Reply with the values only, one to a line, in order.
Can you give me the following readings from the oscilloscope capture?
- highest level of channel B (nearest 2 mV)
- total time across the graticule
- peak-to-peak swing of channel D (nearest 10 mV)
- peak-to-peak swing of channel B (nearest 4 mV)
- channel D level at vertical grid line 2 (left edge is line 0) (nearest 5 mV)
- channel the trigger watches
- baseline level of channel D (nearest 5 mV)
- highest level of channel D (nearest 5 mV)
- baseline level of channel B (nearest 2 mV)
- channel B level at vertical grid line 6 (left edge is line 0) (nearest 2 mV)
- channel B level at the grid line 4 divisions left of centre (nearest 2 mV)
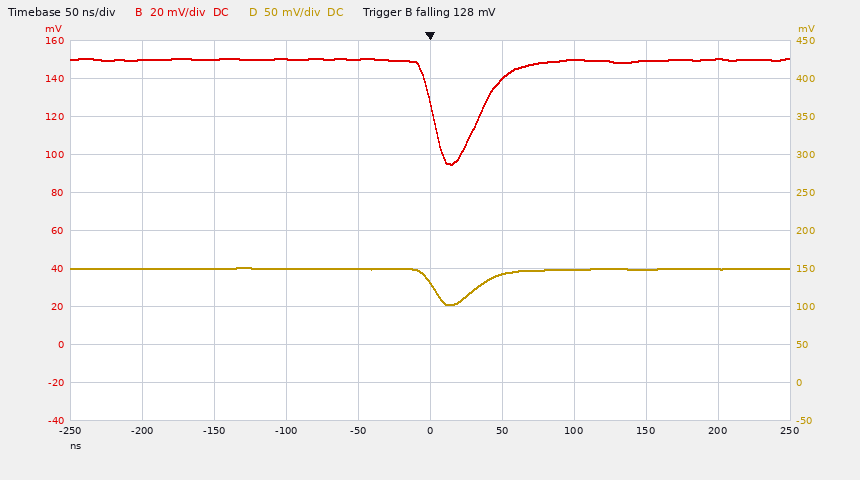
150 mV
500 ns
50 mV
56 mV
150 mV
channel B
150 mV
150 mV
150 mV
140 mV
150 mV
